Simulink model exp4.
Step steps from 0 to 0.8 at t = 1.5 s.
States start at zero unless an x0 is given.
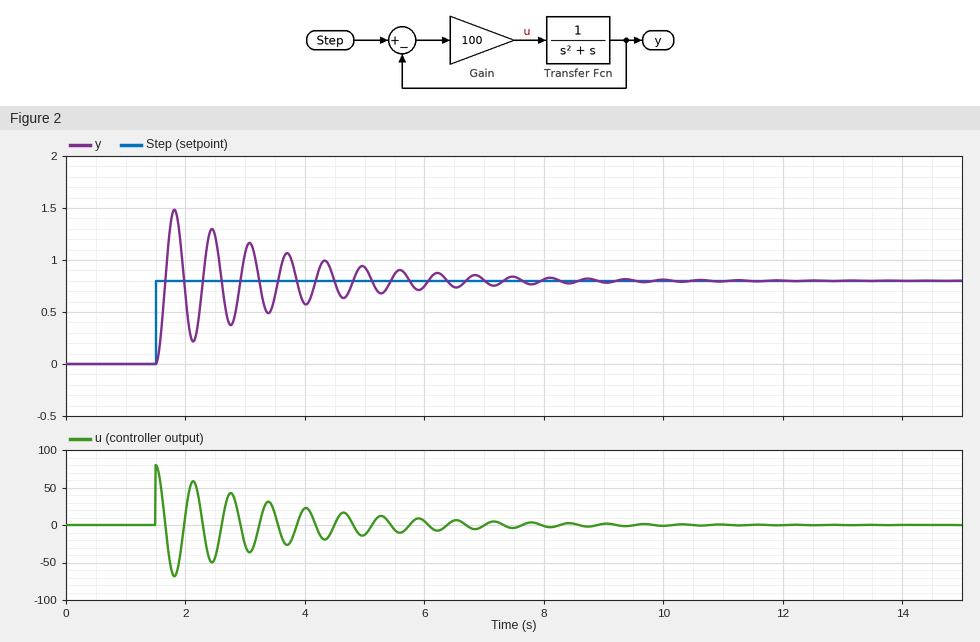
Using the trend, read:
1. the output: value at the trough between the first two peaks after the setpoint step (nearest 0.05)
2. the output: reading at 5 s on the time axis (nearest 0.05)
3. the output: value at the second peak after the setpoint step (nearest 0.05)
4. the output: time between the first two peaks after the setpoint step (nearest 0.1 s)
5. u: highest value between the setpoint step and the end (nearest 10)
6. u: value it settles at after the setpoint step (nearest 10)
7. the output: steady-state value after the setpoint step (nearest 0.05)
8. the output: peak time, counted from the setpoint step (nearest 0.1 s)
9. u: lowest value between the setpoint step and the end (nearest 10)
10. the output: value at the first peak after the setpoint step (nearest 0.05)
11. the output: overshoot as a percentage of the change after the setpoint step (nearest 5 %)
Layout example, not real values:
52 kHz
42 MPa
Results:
0.20
0.95
1.30
0.6 s
80
0
0.80
0.3 s
-70
1.50
85 %
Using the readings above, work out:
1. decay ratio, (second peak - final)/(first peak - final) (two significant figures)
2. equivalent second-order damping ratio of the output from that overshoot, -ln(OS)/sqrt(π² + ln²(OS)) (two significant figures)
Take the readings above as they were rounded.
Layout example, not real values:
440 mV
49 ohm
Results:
0.71
0.052
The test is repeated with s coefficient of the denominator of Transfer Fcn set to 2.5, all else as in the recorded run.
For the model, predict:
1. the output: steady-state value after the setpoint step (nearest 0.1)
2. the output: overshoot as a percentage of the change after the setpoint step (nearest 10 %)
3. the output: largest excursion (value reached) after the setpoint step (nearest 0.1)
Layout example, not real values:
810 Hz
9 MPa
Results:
0.8
70 %
1.3
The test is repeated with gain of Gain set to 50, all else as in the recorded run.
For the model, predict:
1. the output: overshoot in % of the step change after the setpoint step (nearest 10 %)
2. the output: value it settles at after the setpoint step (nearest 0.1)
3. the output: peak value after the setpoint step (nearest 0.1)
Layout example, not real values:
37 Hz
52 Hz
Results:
80 %
0.8
1.4
